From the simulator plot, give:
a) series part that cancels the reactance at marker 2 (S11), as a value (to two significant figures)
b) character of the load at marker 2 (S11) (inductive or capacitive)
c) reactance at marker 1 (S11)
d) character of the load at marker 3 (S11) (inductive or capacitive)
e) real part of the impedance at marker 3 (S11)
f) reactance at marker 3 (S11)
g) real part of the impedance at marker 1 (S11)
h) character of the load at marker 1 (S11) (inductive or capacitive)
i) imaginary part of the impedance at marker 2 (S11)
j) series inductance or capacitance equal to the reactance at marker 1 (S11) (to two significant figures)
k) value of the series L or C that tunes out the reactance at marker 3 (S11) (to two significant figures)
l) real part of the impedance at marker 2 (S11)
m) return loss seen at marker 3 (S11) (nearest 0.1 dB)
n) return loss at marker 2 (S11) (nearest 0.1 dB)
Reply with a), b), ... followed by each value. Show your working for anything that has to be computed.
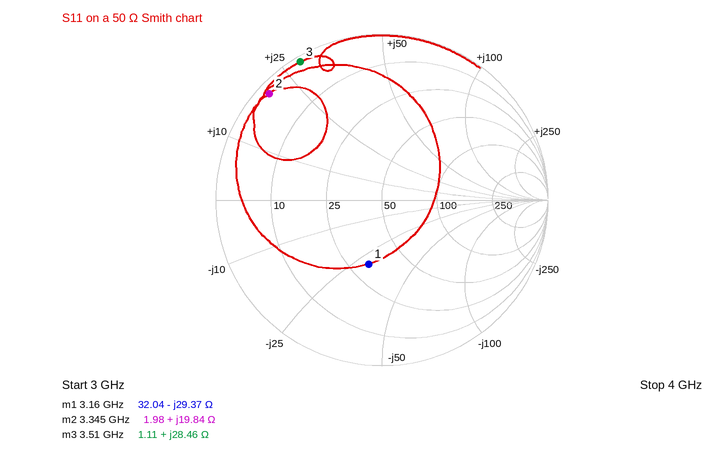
a) C = 1/(2π × 3.345 GHz × 19.84 Ω) ≈ 2.4 pF
b) inductive
c) -29.37 Ω
d) inductive
e) 1.11 Ω
f) +28.46 Ω
g) 32.04 Ω
h) capacitive
i) +19.84 Ω
j) C = 1/(2π × 3.16 GHz × 29.37 Ω) ≈ 1.7 pF
k) C = 1/(2π × 3.51 GHz × 28.46 Ω) ≈ 1.6 pF
l) 1.98 Ω
m) 0.3 dB
n) 0.6 dB
